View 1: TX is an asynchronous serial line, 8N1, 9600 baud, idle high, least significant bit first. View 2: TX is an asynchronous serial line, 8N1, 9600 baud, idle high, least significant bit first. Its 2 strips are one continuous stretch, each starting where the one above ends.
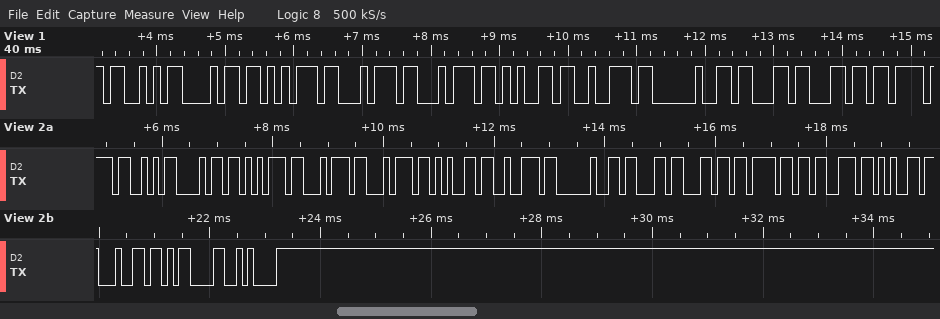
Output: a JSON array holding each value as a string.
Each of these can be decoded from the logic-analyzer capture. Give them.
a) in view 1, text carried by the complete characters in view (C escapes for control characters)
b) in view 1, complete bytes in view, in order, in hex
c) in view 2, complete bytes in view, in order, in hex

["\"Shutter cl\"", "0x53 0x68 0x75 0x74 0x74 0x65 0x72 0x20 0x63 0x6C", "53 68 75 74 74 65 72 20 63 6C 6F 73 65 64 0D 0A"]
